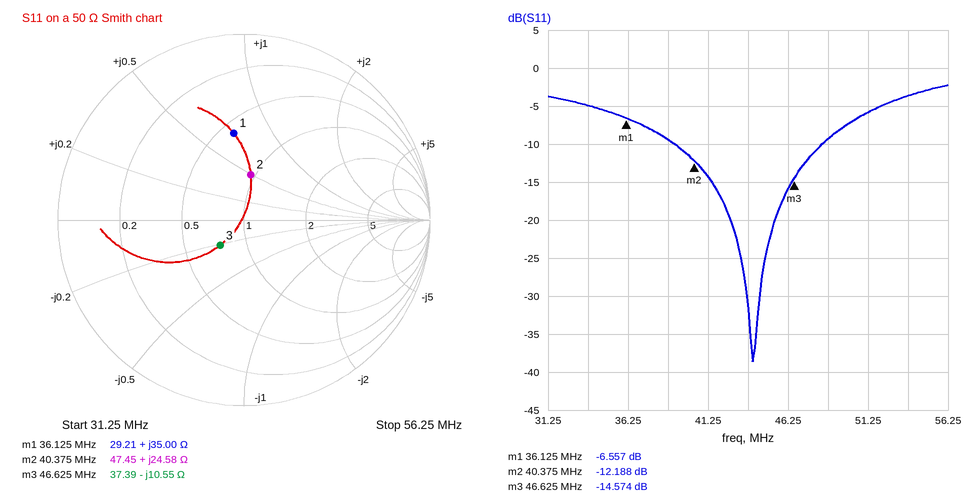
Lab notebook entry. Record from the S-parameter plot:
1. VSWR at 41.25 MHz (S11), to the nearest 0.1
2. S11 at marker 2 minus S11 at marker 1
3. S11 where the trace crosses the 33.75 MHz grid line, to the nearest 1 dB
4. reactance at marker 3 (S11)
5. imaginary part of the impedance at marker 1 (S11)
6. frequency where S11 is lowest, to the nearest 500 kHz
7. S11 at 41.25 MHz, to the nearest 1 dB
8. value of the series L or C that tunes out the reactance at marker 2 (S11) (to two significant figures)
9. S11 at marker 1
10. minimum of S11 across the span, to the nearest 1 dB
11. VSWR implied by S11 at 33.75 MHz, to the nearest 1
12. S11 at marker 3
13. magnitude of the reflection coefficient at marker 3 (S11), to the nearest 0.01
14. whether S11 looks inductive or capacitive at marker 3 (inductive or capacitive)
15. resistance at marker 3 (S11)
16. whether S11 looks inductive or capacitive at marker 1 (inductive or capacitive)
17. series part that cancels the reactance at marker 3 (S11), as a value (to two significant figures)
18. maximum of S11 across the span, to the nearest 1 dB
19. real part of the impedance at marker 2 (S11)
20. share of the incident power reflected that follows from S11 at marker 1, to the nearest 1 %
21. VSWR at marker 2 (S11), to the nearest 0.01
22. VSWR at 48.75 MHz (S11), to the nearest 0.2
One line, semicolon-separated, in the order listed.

1.5; -5.631 dB; -5 dB; -10.55 Ω; +35.00 Ω; 44.0 MHz; -14 dB; 160 pF; -6.557 dB; -39 dB; 4; -14.574 dB; 0.19; capacitive; 37.39 Ω; inductive; 36 nH; -2 dB; 47.45 Ω; 22 %; 1.65; 2.0
